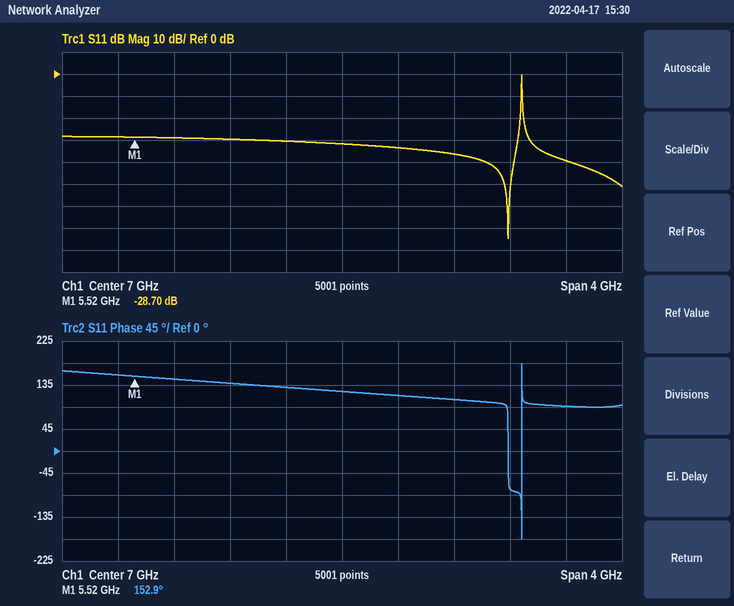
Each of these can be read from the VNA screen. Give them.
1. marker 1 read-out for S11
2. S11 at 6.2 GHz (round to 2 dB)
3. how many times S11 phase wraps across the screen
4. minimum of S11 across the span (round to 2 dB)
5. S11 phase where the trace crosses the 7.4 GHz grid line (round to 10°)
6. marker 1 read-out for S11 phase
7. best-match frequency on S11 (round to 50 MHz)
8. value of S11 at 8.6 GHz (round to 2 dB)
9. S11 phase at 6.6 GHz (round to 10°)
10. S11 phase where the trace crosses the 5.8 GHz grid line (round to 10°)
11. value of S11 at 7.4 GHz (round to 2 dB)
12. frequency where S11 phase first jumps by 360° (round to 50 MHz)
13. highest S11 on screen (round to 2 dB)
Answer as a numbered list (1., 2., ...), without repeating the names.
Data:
1. -28.70 dB
2. -30 dB
3. 1
4. -74 dB
5. 110°
6. 152.9°
7. 8.20 GHz
8. -40 dB
9. 130°
10. 150°
11. -34 dB
12. 8.30 GHz
13. 0 dB
